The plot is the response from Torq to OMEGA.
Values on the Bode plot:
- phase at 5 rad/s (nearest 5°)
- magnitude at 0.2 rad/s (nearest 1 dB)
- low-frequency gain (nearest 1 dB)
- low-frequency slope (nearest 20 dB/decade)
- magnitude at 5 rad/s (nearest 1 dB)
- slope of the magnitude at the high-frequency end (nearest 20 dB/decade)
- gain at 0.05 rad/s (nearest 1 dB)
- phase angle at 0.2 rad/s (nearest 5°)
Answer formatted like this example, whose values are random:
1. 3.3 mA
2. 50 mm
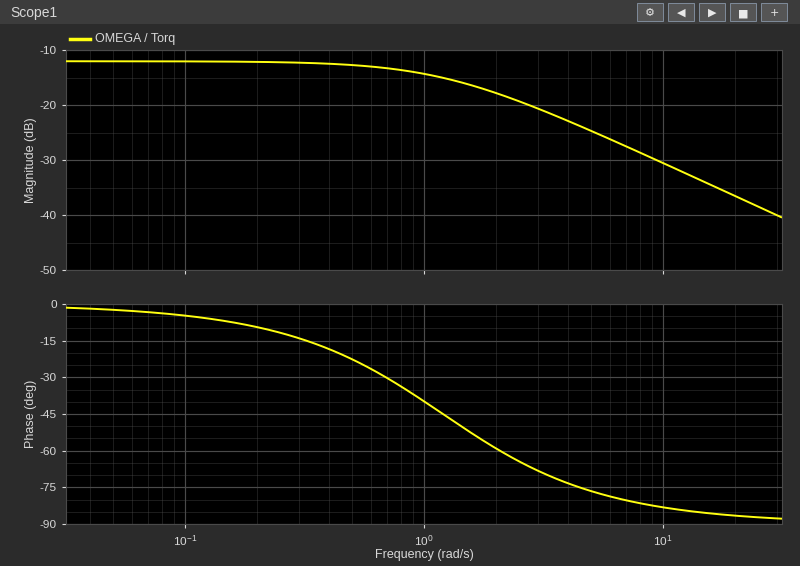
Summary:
1. -75°
2. -12 dB
3. -12 dB
4. 0 dB/decade
5. -25 dB
6. -20 dB/decade
7. -12 dB
8. -10°
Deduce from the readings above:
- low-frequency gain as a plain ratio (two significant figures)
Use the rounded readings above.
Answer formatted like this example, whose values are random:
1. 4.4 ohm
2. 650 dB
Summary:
1. 0.25
